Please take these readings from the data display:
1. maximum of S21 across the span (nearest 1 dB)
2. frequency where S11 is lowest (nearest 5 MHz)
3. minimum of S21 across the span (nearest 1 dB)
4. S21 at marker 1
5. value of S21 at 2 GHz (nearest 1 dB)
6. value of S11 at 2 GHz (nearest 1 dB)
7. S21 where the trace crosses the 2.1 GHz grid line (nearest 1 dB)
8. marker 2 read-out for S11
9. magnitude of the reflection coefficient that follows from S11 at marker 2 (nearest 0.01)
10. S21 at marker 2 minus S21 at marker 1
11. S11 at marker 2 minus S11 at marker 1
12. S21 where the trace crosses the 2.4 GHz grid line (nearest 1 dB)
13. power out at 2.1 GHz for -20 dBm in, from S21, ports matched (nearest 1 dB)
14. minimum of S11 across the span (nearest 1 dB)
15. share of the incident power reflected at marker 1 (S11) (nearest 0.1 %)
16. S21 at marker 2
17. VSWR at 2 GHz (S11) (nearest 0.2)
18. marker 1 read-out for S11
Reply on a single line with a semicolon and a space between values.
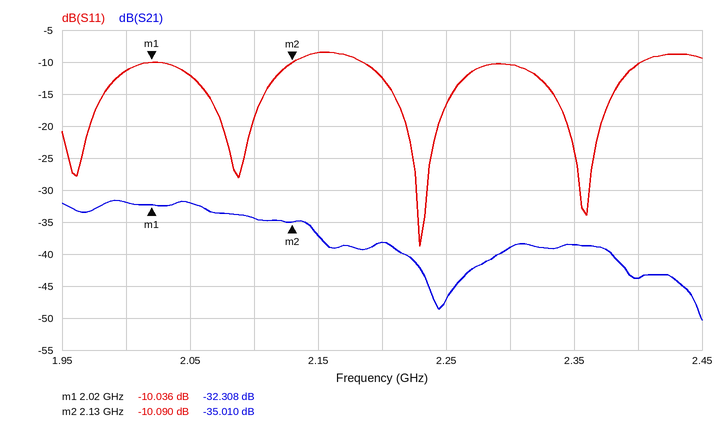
-32 dB; 2.230 GHz; -50 dB; -32.308 dB; -32 dB; -11 dB; -34 dB; -10.090 dB; 0.31; -2.702 dB; -0.054 dB; -44 dB; -54 dBm; -39 dB; 9.9 %; -35.010 dB; 1.8; -10.036 dB
